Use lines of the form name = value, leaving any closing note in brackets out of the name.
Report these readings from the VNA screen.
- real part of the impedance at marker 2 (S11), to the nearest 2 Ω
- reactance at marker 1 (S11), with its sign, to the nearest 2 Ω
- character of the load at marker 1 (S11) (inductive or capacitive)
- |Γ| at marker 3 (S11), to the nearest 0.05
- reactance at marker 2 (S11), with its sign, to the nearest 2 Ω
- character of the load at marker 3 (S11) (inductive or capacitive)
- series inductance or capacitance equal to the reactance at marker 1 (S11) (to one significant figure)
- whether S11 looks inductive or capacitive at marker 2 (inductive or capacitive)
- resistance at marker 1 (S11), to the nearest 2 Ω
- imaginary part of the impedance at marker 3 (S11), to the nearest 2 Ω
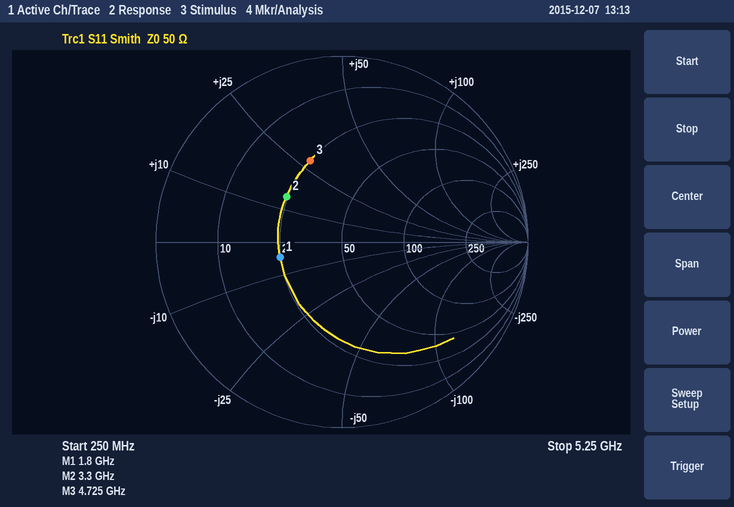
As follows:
real part of the impedance at marker 2 (S11), to the nearest 2 Ω = 24 Ω
reactance at marker 1 (S11), with its sign, to the nearest 2 Ω = -4 Ω
character of the load at marker 1 (S11) = capacitive
|Γ| at marker 3 (S11), to the nearest 0.05 = 0.45
reactance at marker 2 (S11), with its sign, to the nearest 2 Ω = +14 Ω
character of the load at marker 3 (S11) = inductive
series inductance or capacitance equal to the reactance at marker 1 (S11) = 20 pF
whether S11 looks inductive or capacitive at marker 2 = inductive
resistance at marker 1 (S11), to the nearest 2 Ω = 24 Ω
imaginary part of the impedance at marker 3 (S11), to the nearest 2 Ω = +28 Ω
